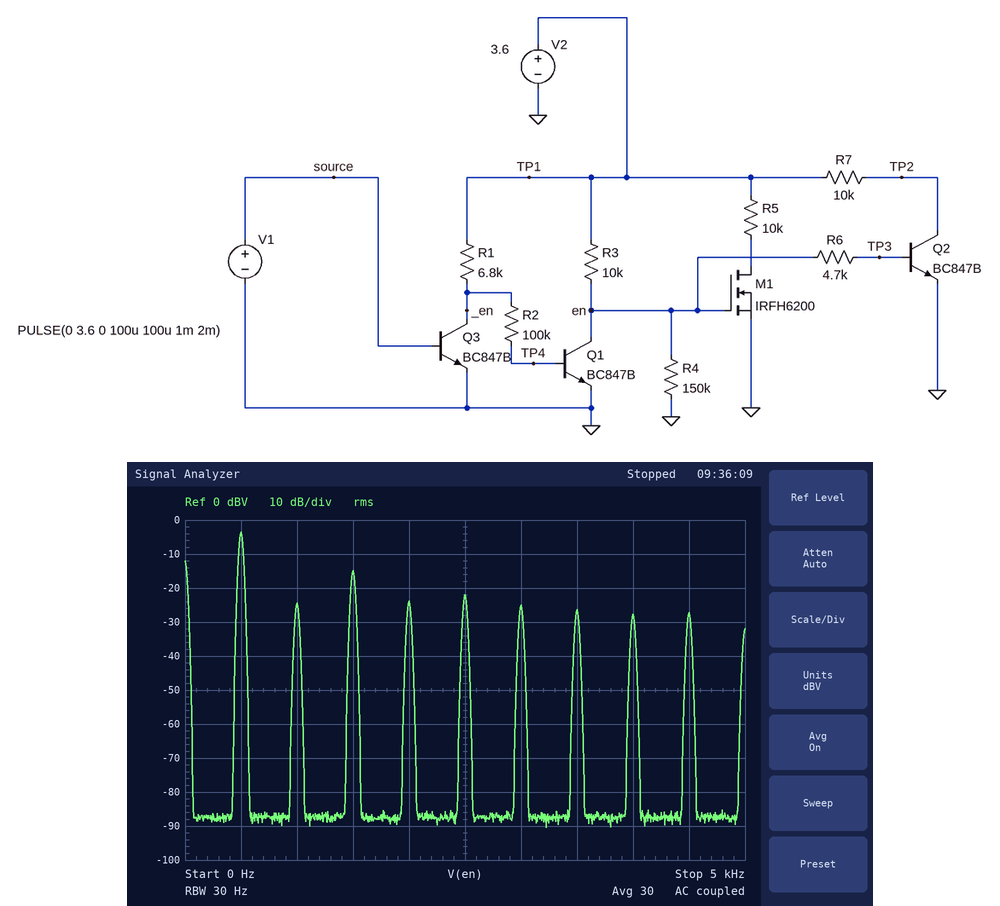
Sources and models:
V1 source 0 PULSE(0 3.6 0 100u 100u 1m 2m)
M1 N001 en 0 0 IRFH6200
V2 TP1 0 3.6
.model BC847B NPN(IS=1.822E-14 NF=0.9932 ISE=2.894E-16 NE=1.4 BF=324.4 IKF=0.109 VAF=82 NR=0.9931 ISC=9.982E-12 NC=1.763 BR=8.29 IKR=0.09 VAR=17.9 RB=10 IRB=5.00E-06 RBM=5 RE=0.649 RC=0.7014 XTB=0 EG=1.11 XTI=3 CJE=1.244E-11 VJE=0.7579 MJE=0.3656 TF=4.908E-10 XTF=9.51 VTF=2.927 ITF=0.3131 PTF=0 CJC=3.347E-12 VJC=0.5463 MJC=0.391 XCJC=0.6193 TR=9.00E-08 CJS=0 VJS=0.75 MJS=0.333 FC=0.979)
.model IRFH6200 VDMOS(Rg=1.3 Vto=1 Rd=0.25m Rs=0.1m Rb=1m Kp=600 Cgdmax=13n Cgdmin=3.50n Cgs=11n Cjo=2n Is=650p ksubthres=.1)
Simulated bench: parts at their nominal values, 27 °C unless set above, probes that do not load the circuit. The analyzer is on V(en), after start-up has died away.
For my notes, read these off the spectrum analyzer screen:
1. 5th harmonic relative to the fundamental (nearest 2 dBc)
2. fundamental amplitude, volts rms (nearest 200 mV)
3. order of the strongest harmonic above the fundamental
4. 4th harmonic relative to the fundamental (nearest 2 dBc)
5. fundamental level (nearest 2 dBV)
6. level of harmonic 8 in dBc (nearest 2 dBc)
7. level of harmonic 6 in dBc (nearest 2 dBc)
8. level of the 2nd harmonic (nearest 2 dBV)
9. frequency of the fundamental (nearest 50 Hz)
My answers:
-18 dBc
600 mV
3
-20 dBc
-4 dBV
-24 dBc
-22 dBc
-24 dBV
500 Hz
